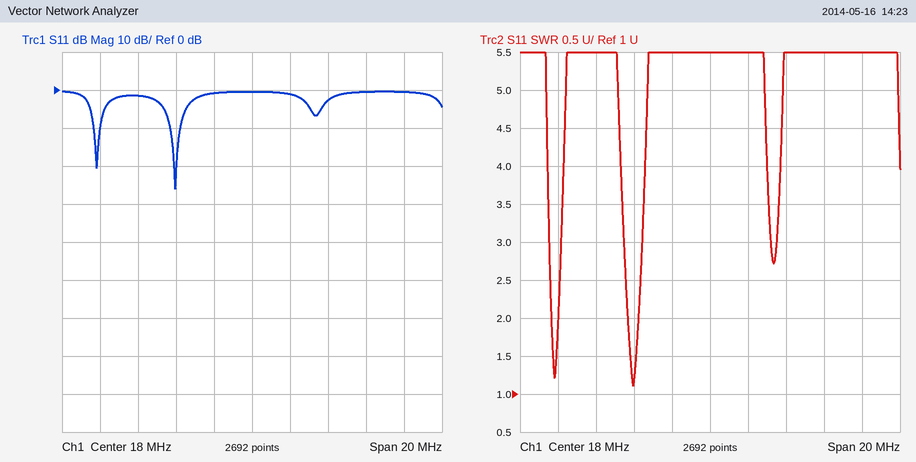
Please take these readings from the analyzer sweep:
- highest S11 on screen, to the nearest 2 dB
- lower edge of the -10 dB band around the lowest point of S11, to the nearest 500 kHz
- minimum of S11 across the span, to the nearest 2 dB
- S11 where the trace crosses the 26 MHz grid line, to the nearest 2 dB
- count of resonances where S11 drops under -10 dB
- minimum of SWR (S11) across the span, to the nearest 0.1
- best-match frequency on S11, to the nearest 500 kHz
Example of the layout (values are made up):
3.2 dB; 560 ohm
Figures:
0 dB; 13.5 MHz; -26 dB; 0 dB; 2; 1.1; 14.0 MHz
